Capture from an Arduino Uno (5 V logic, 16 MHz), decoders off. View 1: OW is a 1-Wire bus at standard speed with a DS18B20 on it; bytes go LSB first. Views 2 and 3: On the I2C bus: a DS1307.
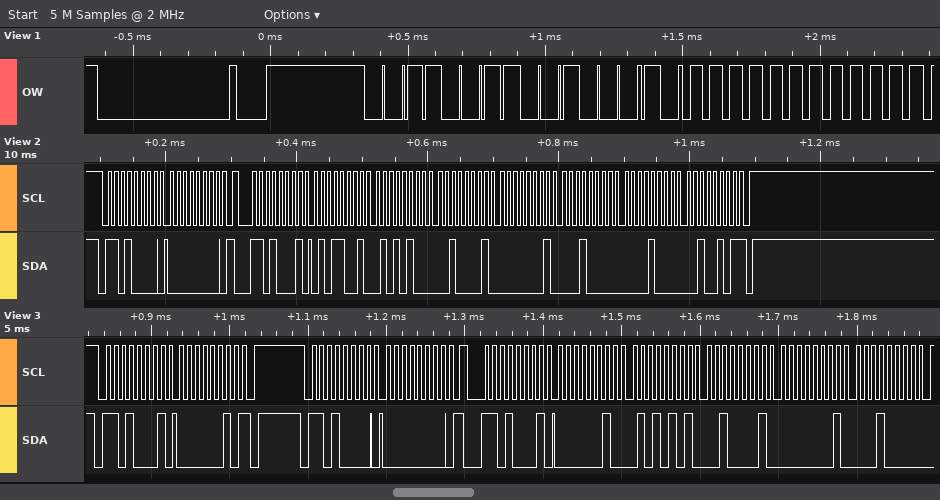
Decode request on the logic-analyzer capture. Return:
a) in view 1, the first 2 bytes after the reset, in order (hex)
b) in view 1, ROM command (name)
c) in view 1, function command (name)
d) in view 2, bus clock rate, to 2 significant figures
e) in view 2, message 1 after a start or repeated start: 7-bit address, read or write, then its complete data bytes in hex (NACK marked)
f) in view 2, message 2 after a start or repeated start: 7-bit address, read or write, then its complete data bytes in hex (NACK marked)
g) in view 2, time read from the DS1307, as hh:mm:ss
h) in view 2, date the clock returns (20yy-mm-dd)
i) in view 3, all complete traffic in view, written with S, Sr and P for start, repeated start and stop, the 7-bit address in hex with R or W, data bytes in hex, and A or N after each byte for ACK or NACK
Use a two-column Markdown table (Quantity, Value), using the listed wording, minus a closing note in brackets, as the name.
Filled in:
| Quantity | Value |
|---|---|
| in view 1, the first 2 bytes after the reset, in order | CC 44 |
| in view 1, ROM command | Skip ROM |
| in view 1, function command | Convert T |
| in view 2, bus clock rate, to 2 significant figures | 100 kHz |
| in view 2, message 1 after a start or repeated start: 7-bit address, read or write, then its complete data bytes in hex | 0x68 write: 00 |
| in view 2, message 2 after a start or repeated start: 7-bit address, read or write, then its complete data bytes in hex | 0x68 read: 59 54 21 01 10 08 25 NACK |
| in view 2, time read from the DS1307, as hh:mm:ss | 21:54:59 |
| in view 2, date the clock returns | 2025-08-10 |
| in view 3, all complete traffic in view, written with S, Sr and P for start, repeated start and stop, the 7-bit address in hex with R or W, data bytes in hex, and A or N after each byte for ACK or NACK | S 68R A 02 N P S 68W A 00 A Sr 68R A 02 A 55 A 21 A 01 A 10 A |
